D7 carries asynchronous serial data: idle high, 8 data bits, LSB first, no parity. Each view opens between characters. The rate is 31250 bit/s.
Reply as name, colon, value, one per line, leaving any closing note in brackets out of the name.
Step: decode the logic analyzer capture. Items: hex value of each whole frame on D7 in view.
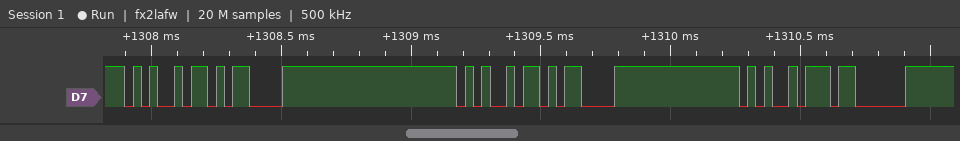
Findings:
hex value of each whole frame on D7 in view: A5, 0D, A5, 0D, A5, 03
